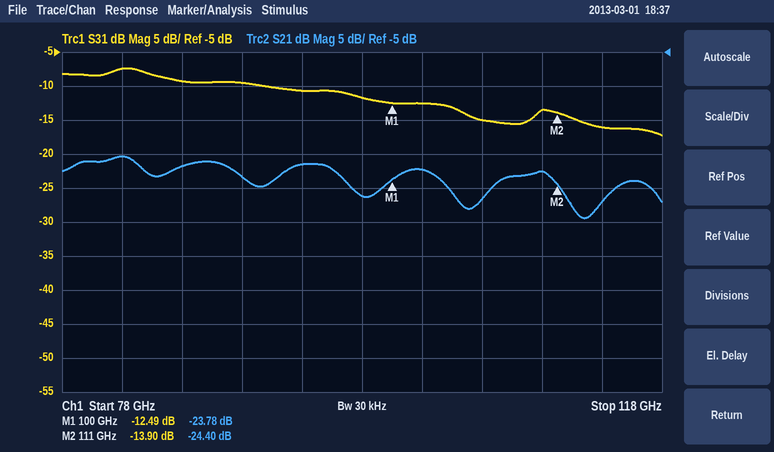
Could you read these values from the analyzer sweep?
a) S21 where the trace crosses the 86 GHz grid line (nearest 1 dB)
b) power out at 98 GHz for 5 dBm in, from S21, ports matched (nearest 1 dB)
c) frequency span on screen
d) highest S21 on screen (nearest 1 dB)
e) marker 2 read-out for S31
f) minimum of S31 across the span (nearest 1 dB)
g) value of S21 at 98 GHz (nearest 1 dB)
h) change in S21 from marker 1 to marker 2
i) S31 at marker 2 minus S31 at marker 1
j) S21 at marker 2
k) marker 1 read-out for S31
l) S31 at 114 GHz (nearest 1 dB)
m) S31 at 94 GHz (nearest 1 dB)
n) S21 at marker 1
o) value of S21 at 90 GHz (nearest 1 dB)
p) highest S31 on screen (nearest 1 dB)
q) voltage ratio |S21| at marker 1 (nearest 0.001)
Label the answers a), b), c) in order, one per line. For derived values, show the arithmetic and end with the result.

a) -22 dB
b) 5 dBm + (-26 dB) = -21 dBm
c) 40 GHz
d) -20 dB
e) -13.90 dB
f) -17 dB
g) -26 dB
h) -24.4 − (-23.78) = -0.62 dB
i) -13.9 − (-12.49) = -1.41 dB
j) -24.40 dB
k) -12.49 dB
l) -16 dB
m) -11 dB
n) -23.78 dB
o) -23 dB
p) -7 dB
q) 10^(-23.78/20) ≈ 0.065
